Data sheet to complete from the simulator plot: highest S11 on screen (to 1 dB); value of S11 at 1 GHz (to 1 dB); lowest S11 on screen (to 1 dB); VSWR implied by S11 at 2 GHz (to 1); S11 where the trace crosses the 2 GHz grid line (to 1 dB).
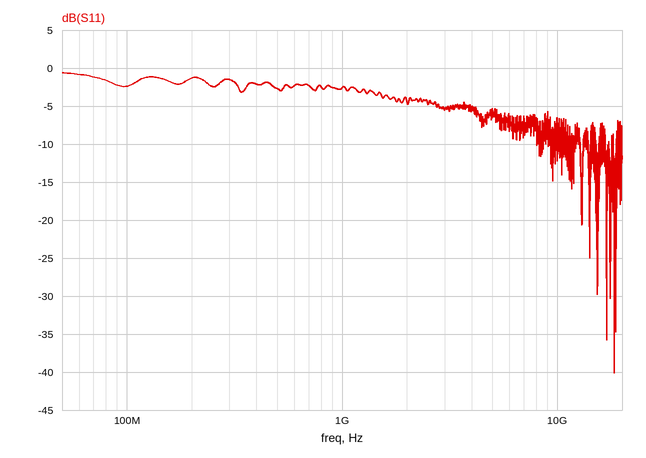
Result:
-1 dB
-3 dB
-40 dB
4
-4 dB
